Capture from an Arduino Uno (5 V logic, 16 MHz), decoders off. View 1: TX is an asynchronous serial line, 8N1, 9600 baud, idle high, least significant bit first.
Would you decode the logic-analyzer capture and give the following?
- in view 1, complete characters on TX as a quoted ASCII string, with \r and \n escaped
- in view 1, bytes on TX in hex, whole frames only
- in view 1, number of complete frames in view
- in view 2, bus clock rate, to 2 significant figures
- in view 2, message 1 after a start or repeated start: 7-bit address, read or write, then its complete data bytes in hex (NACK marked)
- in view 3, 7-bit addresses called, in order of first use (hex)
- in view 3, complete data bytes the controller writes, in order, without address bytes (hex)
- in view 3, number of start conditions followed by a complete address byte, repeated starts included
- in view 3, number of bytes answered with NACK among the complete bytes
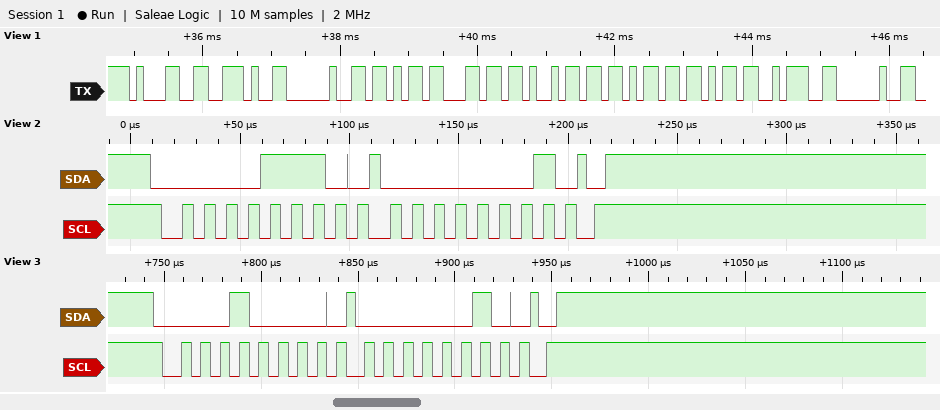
"1. klikk: "
31 2E 20 6B 6C 69 6B 6B 3A 20
10
100 kHz
0x07 write: 01
0x08
02
1
0
